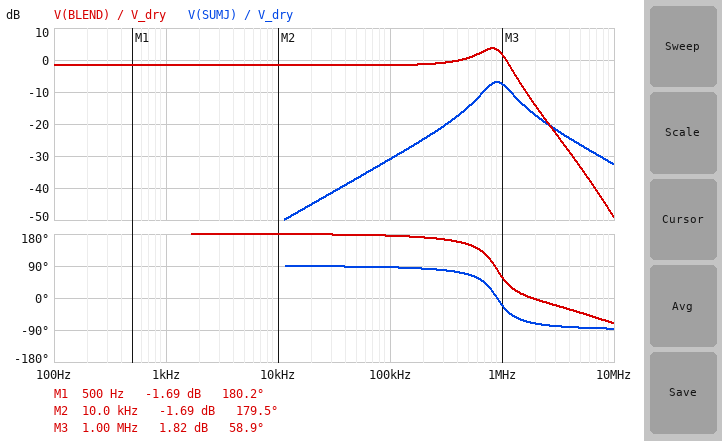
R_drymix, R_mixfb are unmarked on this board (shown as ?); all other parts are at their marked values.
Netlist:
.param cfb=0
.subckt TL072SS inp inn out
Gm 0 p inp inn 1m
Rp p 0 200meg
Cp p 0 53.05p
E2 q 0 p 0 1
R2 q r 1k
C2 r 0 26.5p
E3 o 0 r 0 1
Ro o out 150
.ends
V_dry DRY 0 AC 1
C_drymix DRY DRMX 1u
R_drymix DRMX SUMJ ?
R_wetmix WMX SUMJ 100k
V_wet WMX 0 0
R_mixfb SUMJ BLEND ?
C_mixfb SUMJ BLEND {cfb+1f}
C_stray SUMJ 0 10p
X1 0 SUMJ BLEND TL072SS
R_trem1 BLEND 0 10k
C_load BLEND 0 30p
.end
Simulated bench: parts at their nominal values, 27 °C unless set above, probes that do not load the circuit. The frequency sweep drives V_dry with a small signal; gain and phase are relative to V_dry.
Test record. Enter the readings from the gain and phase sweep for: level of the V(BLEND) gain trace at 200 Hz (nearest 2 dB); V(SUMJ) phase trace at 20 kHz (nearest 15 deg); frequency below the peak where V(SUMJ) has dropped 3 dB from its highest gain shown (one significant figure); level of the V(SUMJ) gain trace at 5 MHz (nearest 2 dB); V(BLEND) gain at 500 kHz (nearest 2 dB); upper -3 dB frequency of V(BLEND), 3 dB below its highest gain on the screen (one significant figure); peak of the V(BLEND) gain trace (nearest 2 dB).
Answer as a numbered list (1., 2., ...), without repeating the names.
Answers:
1. -2 dB
2. 90 deg
3. 700 kHz
4. -26 dB
5. 0 dB
6. 1 MHz
7. 4 dB
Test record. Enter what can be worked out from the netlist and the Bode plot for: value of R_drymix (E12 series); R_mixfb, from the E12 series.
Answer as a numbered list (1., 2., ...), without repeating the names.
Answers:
1. 68 kΩ
2. 56 kΩ
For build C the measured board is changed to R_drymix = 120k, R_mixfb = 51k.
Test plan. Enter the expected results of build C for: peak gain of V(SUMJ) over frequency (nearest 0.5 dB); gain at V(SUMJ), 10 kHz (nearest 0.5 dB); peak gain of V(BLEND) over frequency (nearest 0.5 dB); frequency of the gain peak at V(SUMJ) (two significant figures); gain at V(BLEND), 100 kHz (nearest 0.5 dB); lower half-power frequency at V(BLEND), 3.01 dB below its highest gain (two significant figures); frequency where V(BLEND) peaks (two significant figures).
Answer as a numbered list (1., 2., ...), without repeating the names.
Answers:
1. -10.0 dB
2. -57.0 dB
3. 0 dB
4. 940 kHz
5. -7.5 dB
6. 650 kHz
7. 900 kHz
